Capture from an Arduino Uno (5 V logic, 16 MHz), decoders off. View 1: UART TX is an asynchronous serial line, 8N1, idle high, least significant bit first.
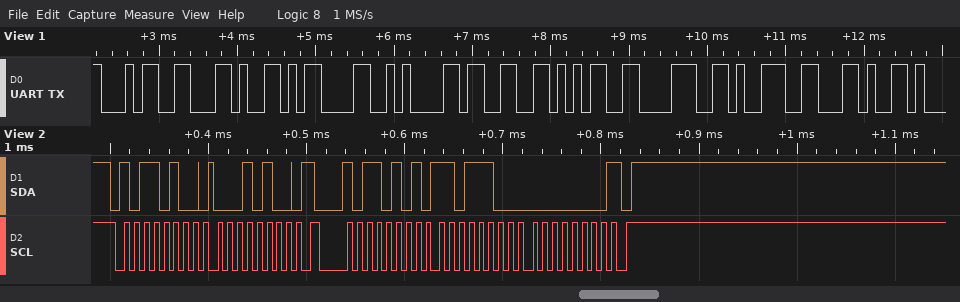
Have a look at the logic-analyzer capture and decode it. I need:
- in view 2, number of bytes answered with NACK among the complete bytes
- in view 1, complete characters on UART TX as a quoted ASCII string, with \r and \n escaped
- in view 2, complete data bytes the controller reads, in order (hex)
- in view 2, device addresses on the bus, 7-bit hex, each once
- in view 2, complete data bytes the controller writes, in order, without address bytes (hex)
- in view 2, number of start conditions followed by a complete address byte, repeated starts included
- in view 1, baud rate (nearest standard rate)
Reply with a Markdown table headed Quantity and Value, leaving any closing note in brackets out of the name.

| Quantity | Value |
|---|---|
| in view 2, number of bytes answered with NACK among the complete bytes | 1 |
| in view 1, complete characters on UART TX as a quoted ASCII string, with \r and \n escaped | "4,\r\n3589," |
| in view 2, complete data bytes the controller reads, in order | DC 00 |
| in view 2, device addresses on the bus, 7-bit hex, each once | 0x5A |
| in view 2, complete data bytes the controller writes, in order, without address bytes | 14 |
| in view 2, number of start conditions followed by a complete address byte, repeated starts included | 2 |
| in view 1, baud rate | 9600 baud |
